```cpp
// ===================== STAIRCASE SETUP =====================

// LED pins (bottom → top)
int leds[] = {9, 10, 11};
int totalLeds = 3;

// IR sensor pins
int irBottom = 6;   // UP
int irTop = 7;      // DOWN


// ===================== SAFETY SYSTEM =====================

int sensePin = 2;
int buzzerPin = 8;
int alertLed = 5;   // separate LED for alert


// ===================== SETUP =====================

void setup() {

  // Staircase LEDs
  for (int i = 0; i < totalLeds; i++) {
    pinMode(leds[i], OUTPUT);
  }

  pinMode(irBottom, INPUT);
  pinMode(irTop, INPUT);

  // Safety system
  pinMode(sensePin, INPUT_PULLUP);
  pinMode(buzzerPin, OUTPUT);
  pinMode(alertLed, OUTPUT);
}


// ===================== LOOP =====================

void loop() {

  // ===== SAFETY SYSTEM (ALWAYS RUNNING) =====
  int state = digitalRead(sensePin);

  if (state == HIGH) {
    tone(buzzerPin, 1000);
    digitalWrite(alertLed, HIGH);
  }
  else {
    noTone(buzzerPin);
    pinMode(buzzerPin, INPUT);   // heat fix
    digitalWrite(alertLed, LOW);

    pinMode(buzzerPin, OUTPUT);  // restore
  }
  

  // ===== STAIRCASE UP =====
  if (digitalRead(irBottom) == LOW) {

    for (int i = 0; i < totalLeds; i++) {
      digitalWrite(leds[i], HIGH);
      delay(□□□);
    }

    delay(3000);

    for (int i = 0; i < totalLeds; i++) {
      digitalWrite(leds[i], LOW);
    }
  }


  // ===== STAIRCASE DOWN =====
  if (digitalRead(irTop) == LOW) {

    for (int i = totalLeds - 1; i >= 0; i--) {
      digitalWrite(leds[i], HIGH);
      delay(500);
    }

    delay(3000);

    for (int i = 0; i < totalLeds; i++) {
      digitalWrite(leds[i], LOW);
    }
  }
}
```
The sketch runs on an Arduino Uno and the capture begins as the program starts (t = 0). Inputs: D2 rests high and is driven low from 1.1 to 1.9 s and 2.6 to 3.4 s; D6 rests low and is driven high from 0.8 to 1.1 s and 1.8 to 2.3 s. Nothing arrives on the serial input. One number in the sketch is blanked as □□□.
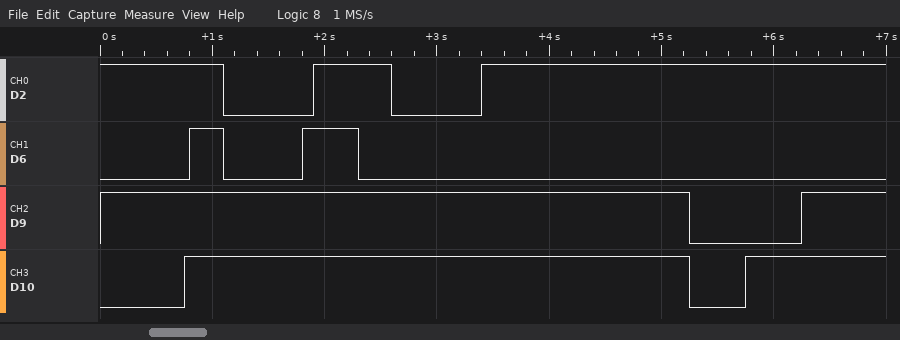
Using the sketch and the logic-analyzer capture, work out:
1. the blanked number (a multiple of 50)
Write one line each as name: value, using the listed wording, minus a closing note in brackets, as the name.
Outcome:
the blanked number: 750
